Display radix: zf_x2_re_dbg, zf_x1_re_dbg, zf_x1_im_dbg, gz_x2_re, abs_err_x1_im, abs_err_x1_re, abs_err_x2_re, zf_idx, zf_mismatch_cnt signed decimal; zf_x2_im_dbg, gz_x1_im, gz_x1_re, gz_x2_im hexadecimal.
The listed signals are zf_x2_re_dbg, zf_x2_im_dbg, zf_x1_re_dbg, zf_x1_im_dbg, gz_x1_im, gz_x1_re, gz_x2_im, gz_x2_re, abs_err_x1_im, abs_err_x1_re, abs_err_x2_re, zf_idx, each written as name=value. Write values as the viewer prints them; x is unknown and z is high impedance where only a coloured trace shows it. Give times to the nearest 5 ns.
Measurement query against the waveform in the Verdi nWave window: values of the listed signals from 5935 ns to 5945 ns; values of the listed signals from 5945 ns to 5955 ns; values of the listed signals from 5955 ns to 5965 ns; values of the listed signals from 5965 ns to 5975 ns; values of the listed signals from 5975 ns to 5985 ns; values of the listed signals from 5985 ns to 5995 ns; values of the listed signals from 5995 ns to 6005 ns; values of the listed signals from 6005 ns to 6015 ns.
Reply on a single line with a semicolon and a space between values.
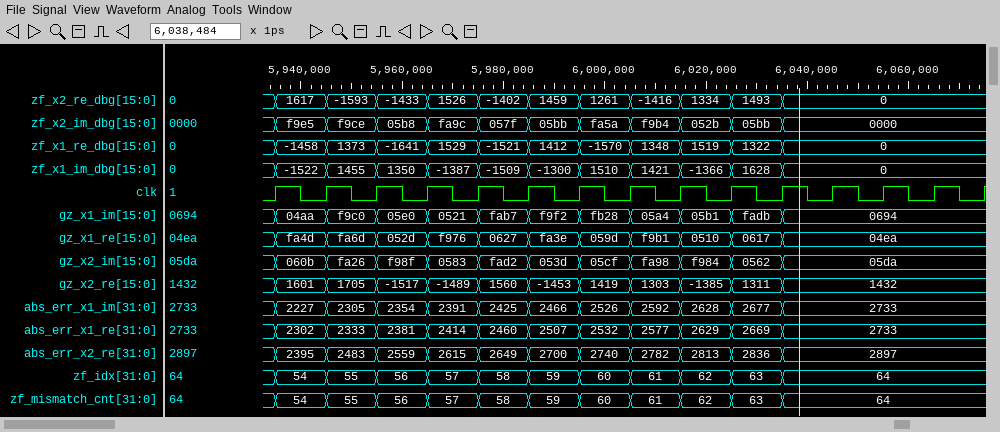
zf_x2_re_dbg=1617, zf_x2_im_dbg=f9e5, zf_x1_re_dbg=-1458, zf_x1_im_dbg=-1522, gz_x1_im=04aa, gz_x1_re=fa4d, gz_x2_im=060b, gz_x2_re=1601, abs_err_x1_im=2227, abs_err_x1_re=2302, abs_err_x2_re=2395, zf_idx=54; zf_x2_re_dbg=-1593, zf_x2_im_dbg=f9ce, zf_x1_re_dbg=1373, zf_x1_im_dbg=1455, gz_x1_im=f9c0, gz_x1_re=fa6d, gz_x2_im=fa26, gz_x2_re=1705, abs_err_x1_im=2305, abs_err_x1_re=2333, abs_err_x2_re=2483, zf_idx=55; zf_x2_re_dbg=-1433, zf_x2_im_dbg=05b8, zf_x1_re_dbg=-1641, zf_x1_im_dbg=1350, gz_x1_im=05e0, gz_x1_re=052d, gz_x2_im=f98f, gz_x2_re=-1517, abs_err_x1_im=2354, abs_err_x1_re=2381, abs_err_x2_re=2559, zf_idx=56; zf_x2_re_dbg=1526, zf_x2_im_dbg=fa9c, zf_x1_re_dbg=1529, zf_x1_im_dbg=-1387, gz_x1_im=0521, gz_x1_re=f976, gz_x2_im=0583, gz_x2_re=-1489, abs_err_x1_im=2391, abs_err_x1_re=2414, abs_err_x2_re=2615, zf_idx=57; zf_x2_re_dbg=-1402, zf_x2_im_dbg=057f, zf_x1_re_dbg=-1521, zf_x1_im_dbg=-1509, gz_x1_im=fab7, gz_x1_re=0627, gz_x2_im=fad2, gz_x2_re=1560, abs_err_x1_im=2425, abs_err_x1_re=2460, abs_err_x2_re=2649, zf_idx=58; zf_x2_re_dbg=1459, zf_x2_im_dbg=05bb, zf_x1_re_dbg=1412, zf_x1_im_dbg=-1300, gz_x1_im=f9f2, gz_x1_re=fa3e, gz_x2_im=053d, gz_x2_re=-1453, abs_err_x1_im=2466, abs_err_x1_re=2507, abs_err_x2_re=2700, zf_idx=59; zf_x2_re_dbg=1261, zf_x2_im_dbg=fa5a, zf_x1_re_dbg=-1570, zf_x1_im_dbg=1510, gz_x1_im=fb28, gz_x1_re=059d, gz_x2_im=05cf, gz_x2_re=1419, abs_err_x1_im=2526, abs_err_x1_re=2532, abs_err_x2_re=2740, zf_idx=60; zf_x2_re_dbg=-1416, zf_x2_im_dbg=f9b4, zf_x1_re_dbg=1348, zf_x1_im_dbg=1421, gz_x1_im=05a4, gz_x1_re=f9b1, gz_x2_im=fa98, gz_x2_re=1303, abs_err_x1_im=2592, abs_err_x1_re=2577, abs_err_x2_re=2782, zf_idx=61
